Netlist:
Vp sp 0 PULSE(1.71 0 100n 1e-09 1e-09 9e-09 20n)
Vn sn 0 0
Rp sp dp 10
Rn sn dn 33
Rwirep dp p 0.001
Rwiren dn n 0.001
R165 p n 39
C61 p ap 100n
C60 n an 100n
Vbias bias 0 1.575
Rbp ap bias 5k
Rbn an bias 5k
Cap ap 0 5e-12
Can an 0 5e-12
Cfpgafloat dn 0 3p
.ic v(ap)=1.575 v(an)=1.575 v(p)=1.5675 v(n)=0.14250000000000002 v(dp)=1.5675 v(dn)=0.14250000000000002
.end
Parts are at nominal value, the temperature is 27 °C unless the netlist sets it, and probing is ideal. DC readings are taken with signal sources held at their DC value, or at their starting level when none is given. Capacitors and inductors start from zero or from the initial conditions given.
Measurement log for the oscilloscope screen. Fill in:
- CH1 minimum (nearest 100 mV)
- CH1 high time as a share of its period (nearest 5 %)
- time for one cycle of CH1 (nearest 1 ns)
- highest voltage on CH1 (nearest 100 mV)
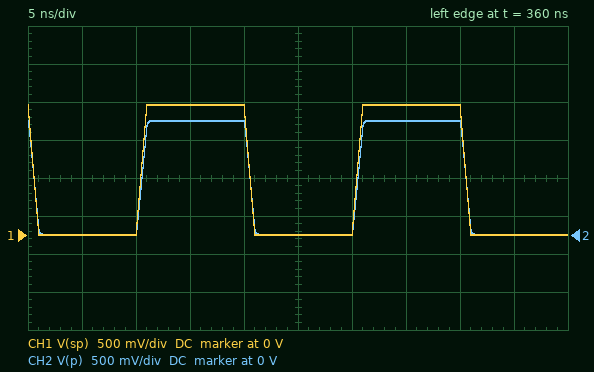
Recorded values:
0 V
50 %
20 ns
1.7 V
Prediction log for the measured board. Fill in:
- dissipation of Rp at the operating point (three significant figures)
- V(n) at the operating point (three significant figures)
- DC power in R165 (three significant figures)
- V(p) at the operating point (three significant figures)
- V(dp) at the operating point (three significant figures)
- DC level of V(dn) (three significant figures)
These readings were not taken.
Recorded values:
4.35 mW
688 mV
17.0 mW
1.50 V
1.50 V
688 mV
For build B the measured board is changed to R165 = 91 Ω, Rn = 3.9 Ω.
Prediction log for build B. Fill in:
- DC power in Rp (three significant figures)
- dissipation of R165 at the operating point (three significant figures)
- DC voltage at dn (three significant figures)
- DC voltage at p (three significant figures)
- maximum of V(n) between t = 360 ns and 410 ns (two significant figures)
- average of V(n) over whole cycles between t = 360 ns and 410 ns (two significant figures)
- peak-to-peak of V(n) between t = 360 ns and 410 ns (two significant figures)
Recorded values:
2.66 mW
24.2 mW
63.6 mV
1.55 V
64 mV
32 mV
63 mV
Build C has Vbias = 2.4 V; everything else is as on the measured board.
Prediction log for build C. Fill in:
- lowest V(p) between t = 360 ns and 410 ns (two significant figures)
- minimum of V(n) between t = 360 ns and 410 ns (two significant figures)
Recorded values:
5.0 mV
5.7 mV
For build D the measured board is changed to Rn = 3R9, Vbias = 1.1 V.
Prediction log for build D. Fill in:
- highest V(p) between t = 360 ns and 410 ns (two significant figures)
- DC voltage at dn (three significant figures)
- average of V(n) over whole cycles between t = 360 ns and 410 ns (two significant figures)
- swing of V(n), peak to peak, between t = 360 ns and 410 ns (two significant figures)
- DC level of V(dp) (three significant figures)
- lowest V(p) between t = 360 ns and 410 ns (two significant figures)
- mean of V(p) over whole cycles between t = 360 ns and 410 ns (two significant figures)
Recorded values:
1.4 V
126 mV
63 mV
130 mV
1.39 V
1.7 mV
690 mV
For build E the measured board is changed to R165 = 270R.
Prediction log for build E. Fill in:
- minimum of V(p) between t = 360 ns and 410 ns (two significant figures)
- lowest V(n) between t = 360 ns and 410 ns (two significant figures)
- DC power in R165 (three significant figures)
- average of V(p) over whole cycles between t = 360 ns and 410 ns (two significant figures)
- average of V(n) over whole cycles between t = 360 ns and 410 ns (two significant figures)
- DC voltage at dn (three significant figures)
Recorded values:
3.1 mV
1.2 mV
8.06 mW
830 mV
91 mV
180 mV
